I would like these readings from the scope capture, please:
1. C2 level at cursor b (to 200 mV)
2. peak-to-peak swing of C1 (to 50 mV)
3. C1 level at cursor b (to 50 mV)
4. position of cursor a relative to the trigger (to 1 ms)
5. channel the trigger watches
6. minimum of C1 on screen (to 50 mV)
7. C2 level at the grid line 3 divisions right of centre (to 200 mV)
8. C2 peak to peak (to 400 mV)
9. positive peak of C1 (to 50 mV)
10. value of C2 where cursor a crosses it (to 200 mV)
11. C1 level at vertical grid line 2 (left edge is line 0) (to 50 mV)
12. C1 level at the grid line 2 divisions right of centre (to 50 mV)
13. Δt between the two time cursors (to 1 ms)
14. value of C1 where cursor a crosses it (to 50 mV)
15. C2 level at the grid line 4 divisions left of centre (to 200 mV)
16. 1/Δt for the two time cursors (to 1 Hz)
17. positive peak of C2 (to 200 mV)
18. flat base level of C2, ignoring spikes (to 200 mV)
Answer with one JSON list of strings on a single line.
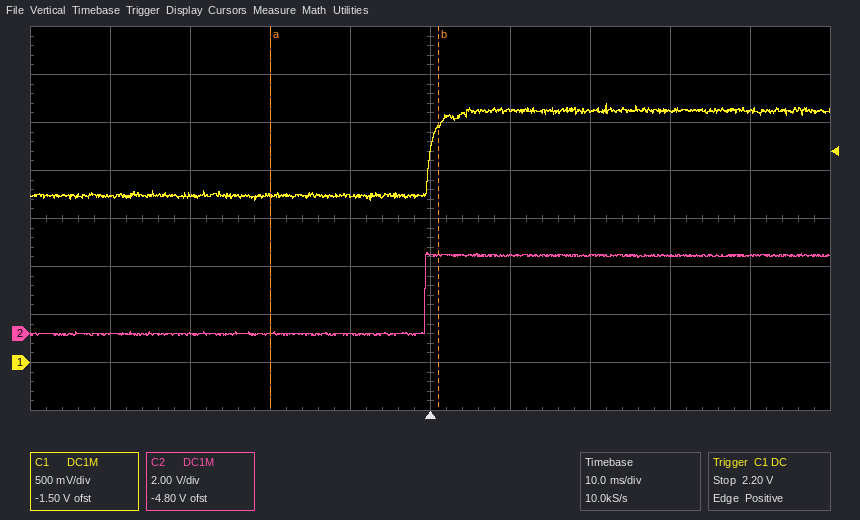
["3.2 V", "1.00 V", "2.45 V", "-20 ms", "C1", "1.70 V", "3.2 V", "3.6 V", "2.70 V", "0.0 V", "1.75 V", "2.60 V", "21 ms", "1.75 V", "0.0 V", "48 Hz", "3.4 V", "0.0 V"]
